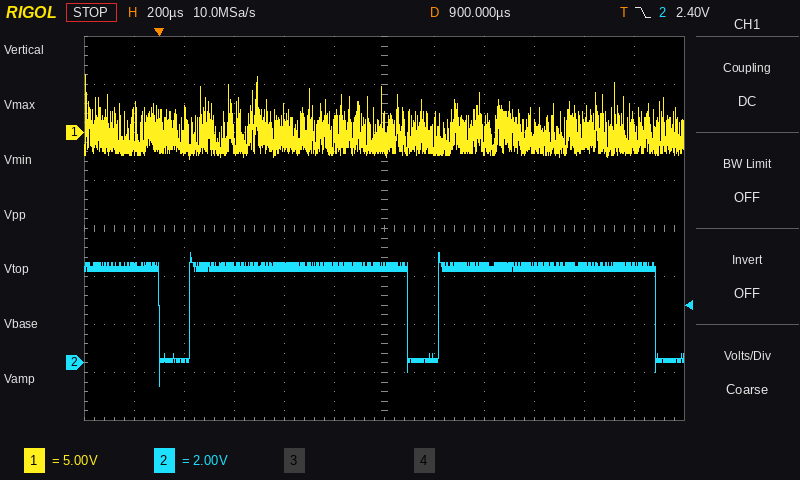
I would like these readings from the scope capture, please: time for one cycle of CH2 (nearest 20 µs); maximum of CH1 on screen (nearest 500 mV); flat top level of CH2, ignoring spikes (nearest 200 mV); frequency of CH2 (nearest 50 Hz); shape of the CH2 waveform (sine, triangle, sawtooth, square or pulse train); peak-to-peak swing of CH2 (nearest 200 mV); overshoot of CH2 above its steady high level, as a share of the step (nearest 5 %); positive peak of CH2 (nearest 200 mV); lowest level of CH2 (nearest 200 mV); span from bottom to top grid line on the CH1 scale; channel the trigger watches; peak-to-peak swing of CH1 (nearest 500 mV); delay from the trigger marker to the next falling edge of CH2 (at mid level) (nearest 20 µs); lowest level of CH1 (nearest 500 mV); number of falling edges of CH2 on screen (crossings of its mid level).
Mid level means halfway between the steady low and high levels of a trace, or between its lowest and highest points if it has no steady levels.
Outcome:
1.00 ms
6.0 V
4.0 V
1.00 kHz
pulse train
5.6 V
15 %
4.6 V
-1.0 V
40 V
CH2
9.0 V
1.00 ms
-3.0 V
3
